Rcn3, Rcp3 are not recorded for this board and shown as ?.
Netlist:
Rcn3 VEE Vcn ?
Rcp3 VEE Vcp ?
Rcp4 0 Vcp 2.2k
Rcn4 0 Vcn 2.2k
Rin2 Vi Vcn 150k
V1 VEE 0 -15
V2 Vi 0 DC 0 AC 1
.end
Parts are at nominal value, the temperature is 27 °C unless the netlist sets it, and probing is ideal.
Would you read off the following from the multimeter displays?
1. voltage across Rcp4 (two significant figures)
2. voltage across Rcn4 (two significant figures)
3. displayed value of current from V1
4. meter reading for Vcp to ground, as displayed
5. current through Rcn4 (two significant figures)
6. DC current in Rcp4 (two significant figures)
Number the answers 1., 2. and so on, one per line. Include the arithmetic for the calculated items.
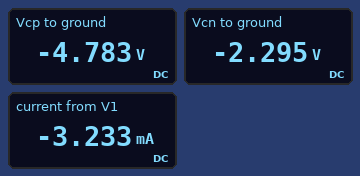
1. 0 V - (-4.783 V) = 4.8 V
2. 0 V - (-2.295 V) = 2.3 V
3. -3.233 mA
4. -4.783 V
5. (0 V - (-2.295 V)) / 2.2 kΩ = 1.0 mA
6. (0 V - (-4.783 V)) / 2.2 kΩ = 2.2 mA
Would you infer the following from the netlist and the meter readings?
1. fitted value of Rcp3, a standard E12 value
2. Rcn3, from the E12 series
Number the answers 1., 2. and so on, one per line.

1. 4.7 kΩ
2. 12 kΩ
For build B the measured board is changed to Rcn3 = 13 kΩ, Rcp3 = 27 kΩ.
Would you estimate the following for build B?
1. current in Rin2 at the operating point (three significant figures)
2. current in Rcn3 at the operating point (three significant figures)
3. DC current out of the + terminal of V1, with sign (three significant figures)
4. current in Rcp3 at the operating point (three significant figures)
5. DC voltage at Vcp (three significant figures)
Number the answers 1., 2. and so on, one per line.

1. 14.3 µA
2. 989 µA
3. -1.50 mA
4. 514 µA
5. -1.13 V
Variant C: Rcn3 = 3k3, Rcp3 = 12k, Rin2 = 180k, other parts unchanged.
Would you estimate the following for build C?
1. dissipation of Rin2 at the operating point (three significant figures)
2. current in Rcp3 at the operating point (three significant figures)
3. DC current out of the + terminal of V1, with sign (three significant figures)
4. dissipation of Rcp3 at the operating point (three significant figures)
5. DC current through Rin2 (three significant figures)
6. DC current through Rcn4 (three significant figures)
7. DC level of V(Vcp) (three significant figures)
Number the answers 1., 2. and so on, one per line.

1. 197 µW
2. 1.06 mA
3. -3.80 mA
4. 13.4 mW
5. 33.1 µA
6. 2.71 mA
7. -2.32 V
